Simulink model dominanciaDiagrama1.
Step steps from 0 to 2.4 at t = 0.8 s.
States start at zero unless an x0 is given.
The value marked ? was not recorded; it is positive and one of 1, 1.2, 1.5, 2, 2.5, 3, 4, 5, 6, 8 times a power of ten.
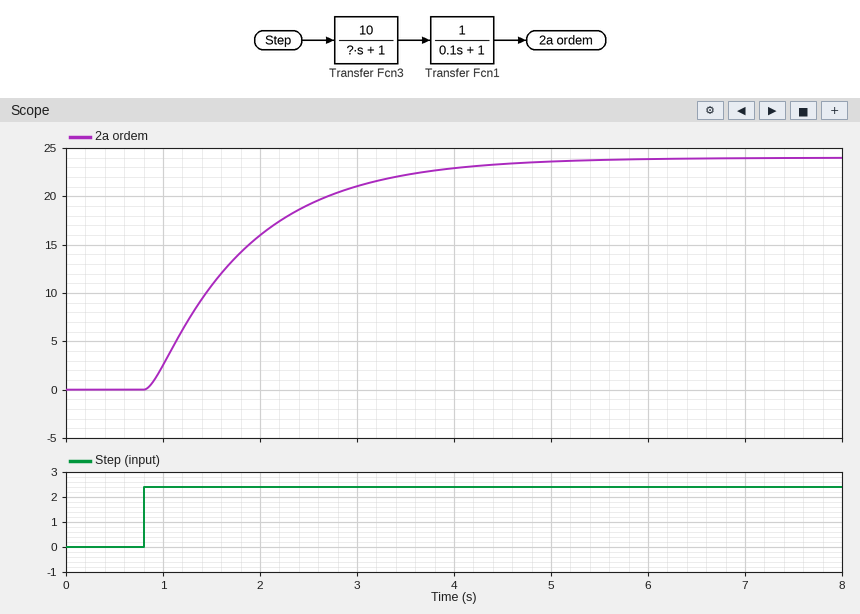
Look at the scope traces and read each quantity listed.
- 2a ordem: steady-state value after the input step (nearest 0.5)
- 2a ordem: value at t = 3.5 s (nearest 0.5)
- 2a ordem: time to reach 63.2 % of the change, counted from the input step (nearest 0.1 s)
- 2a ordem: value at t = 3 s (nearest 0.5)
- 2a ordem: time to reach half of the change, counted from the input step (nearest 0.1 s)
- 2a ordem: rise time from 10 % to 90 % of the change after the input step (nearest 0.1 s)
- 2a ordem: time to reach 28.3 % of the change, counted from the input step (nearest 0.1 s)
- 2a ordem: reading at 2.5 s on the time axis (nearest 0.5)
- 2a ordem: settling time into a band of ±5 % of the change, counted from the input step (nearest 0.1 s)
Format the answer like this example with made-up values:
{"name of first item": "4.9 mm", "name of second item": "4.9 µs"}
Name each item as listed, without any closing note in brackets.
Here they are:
{"2a ordem: steady-state value after the input step": "24.0", "2a ordem: value at t = 3.5 s": "22.0", "2a ordem: time to reach 63.2 % of the change, counted from the input step": "1.1 s", "2a ordem: value at t = 3 s": "21.0", "2a ordem: time to reach half of the change, counted from the input step": "0.8 s", "2a ordem: rise time from 10 % to 90 % of the change after the input step": "2.2 s", "2a ordem: time to reach 28.3 % of the change, counted from the input step": "0.4 s", "2a ordem: reading at 2.5 s on the time axis": "19.0", "2a ordem: settling time into a band of ±5 % of the change, counted from the input step": "3.1 s"}
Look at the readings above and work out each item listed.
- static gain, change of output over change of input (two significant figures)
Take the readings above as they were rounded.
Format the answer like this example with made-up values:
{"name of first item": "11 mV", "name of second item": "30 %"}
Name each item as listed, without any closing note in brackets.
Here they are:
{"static gain, change of output over change of input": "10"}
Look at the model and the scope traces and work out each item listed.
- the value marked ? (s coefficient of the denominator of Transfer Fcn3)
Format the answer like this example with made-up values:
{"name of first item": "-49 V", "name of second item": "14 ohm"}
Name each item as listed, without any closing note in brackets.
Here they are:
{"the value marked ?": "1"}
